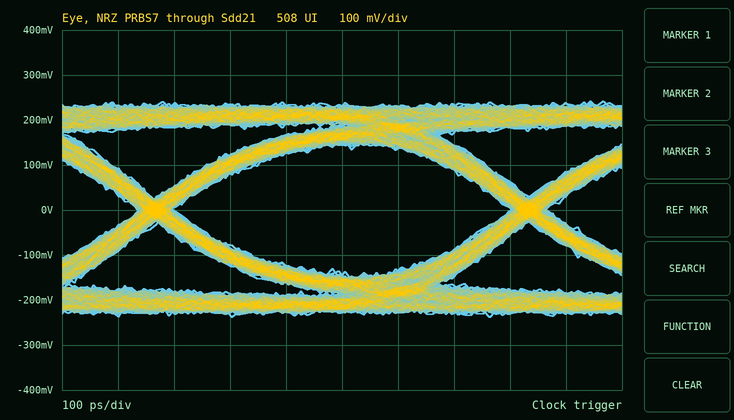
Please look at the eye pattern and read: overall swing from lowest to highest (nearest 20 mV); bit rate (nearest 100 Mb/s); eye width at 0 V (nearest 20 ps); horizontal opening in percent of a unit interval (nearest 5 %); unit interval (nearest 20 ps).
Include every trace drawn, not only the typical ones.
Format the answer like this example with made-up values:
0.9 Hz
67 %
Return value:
480 mV
1.5 Gb/s
600 ps
90 %
660 ps
